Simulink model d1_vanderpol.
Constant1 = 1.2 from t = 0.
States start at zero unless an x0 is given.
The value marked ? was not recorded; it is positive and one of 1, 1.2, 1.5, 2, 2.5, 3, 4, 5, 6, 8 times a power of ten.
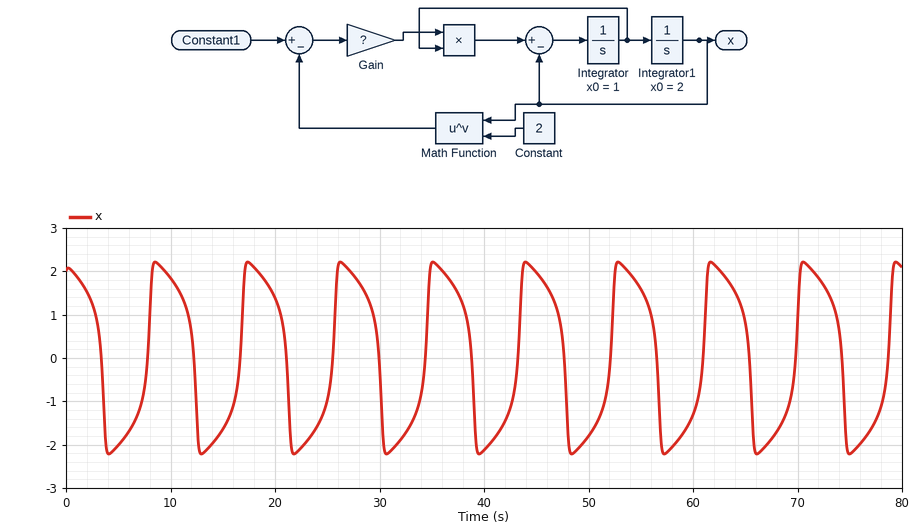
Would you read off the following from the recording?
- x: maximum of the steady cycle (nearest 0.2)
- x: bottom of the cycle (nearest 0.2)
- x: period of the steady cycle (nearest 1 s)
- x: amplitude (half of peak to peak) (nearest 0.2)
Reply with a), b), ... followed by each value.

a) 2.2
b) -2.2
c) 9 s
d) 2.2
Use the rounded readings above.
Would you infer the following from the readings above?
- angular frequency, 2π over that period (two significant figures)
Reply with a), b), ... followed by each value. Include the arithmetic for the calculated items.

a) 2π / 9 = 0.70 rad/s
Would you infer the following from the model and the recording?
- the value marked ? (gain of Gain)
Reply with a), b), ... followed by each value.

a) 2.5
